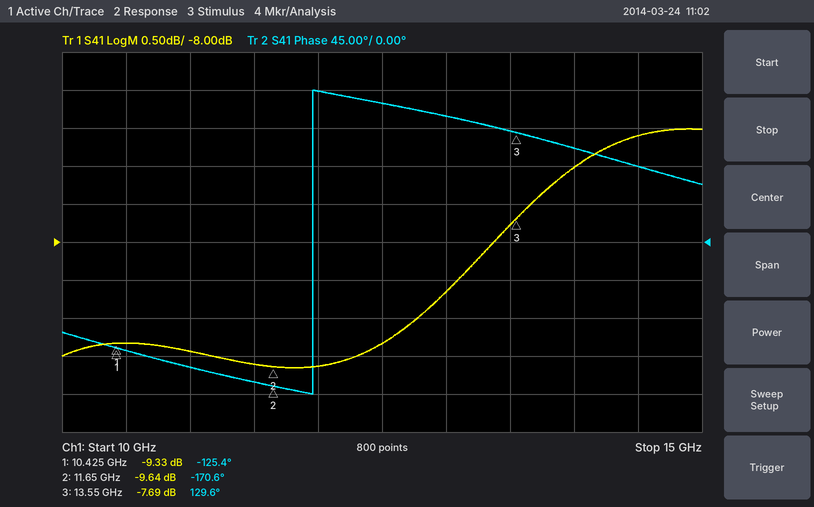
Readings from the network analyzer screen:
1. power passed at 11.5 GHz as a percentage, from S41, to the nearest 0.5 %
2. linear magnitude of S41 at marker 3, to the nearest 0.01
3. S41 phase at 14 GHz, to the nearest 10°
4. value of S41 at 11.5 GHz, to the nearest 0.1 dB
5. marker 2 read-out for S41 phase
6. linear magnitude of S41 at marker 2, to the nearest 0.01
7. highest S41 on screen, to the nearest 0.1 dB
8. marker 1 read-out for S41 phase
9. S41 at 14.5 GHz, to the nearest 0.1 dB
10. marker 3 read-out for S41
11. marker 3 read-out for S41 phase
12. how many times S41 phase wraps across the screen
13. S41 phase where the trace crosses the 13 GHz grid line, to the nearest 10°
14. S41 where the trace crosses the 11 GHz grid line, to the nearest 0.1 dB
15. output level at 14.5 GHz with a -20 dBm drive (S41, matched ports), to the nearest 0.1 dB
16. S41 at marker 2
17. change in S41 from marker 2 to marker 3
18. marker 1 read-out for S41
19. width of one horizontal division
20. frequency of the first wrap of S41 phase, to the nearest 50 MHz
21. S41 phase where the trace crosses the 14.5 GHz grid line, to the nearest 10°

11.0 %
0.41
110°
-9.6 dB
-170.6°
0.33
-6.5 dB
-125.4°
-6.6 dB
-7.69 dB
129.6°
1
150°
-9.4 dB
-26.6 dBm
-9.64 dB
1.95 dB
-9.33 dB
500 MHz
11.95 GHz
90°
